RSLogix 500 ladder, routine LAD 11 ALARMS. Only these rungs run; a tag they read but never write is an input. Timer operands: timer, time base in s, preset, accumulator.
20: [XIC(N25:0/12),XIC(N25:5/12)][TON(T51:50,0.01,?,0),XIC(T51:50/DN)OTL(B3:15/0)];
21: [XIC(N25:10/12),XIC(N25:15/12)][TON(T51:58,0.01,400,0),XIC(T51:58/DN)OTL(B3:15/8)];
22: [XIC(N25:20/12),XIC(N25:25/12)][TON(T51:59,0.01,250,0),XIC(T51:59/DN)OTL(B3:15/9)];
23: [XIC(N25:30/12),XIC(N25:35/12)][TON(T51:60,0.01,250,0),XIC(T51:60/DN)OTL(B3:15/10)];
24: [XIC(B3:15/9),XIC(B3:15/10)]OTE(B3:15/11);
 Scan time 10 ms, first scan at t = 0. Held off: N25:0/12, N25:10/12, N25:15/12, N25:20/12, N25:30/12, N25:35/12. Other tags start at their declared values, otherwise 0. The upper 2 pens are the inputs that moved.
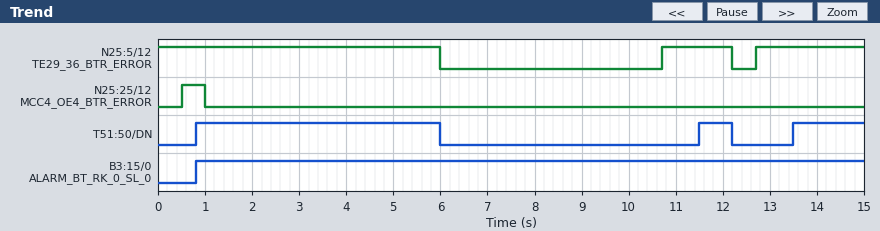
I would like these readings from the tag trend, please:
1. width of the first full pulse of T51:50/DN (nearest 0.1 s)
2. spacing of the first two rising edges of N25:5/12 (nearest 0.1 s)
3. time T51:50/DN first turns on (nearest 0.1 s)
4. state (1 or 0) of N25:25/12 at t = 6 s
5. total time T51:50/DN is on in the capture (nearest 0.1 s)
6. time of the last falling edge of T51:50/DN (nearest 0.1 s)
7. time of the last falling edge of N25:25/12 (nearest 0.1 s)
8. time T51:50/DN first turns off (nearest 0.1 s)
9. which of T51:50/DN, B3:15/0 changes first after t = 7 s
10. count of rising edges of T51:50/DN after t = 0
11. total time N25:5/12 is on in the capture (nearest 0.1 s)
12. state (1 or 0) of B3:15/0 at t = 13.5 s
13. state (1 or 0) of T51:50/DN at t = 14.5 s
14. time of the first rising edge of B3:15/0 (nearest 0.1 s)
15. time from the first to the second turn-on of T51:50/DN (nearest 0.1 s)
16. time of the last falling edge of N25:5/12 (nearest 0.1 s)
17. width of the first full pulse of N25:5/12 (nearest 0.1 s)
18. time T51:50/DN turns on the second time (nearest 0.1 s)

5.2 s
2.0 s
0.8 s
0
7.4 s
12.2 s
1.0 s
6.0 s
T51:50/DN
3
9.8 s
1
1
0.8 s
10.7 s
12.2 s
1.5 s
11.5 s
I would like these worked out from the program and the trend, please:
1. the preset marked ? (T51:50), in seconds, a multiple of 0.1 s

0.8 s
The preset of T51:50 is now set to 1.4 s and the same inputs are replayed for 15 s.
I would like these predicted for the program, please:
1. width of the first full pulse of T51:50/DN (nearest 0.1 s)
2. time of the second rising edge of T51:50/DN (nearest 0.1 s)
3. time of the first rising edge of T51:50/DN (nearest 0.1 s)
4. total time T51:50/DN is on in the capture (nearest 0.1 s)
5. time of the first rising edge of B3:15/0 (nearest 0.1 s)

4.6 s
12.1 s
1.4 s
5.6 s
1.4 s
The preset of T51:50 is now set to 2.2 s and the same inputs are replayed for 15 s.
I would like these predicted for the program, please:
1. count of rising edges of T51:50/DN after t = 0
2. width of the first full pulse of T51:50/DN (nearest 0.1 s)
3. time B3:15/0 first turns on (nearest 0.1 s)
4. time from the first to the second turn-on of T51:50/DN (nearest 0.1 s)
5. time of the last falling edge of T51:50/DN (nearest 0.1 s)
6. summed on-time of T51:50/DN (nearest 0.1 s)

2
3.8 s
2.2 s
12.7 s
6.0 s
3.9 s
